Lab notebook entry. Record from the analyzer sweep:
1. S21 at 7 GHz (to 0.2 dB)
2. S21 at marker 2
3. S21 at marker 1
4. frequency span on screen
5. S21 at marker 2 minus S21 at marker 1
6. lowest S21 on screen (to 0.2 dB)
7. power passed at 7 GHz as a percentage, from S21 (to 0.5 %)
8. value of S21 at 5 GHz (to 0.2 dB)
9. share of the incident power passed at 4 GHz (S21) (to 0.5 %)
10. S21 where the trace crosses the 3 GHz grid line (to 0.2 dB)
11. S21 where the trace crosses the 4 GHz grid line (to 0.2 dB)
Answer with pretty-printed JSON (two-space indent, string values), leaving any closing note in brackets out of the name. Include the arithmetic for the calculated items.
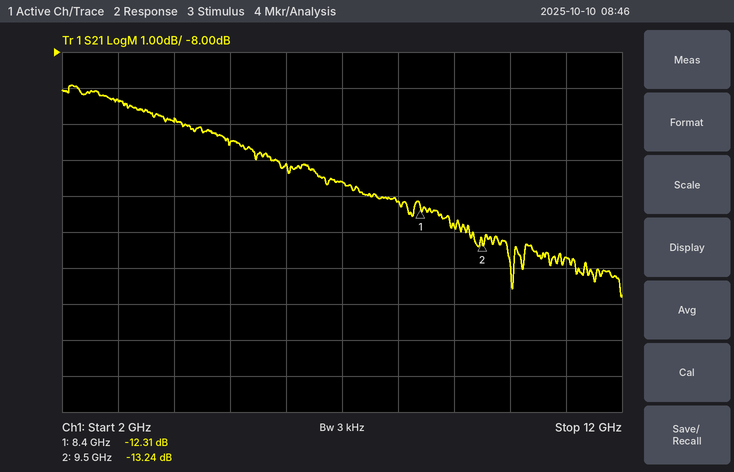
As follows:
{
  "S21 at 7 GHz": "-11.6 dB",
  "S21 at marker 2": "-13.24 dB",
  "S21 at marker 1": "-12.31 dB",
  "frequency span on screen": "10 GHz",
  "S21 at marker 2 minus S21 at marker 1": "-13.24 − (-12.31) = -0.93 dB",
  "lowest S21 on screen": "-14.8 dB",
  "power passed at 7 GHz as a percentage, from S21": "10^(-11.6/10) ≈ 6.92 %, so 7.0 % to the nearest 0.5 %",
  "value of S21 at 5 GHz": "-10.6 dB",
  "share of the incident power passed at 4 GHz (S21)": "10^(-10/10) ≈ 10.0 %",
  "S21 where the trace crosses the 3 GHz grid line": "-9.4 dB",
  "S21 where the trace crosses the 4 GHz grid line": "-10.0 dB"
}
